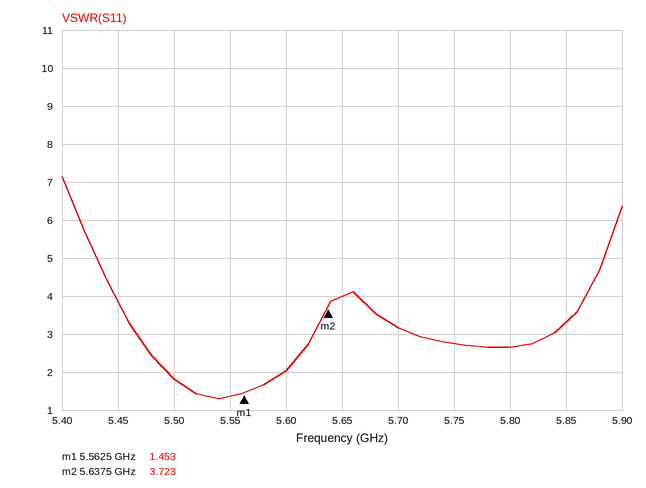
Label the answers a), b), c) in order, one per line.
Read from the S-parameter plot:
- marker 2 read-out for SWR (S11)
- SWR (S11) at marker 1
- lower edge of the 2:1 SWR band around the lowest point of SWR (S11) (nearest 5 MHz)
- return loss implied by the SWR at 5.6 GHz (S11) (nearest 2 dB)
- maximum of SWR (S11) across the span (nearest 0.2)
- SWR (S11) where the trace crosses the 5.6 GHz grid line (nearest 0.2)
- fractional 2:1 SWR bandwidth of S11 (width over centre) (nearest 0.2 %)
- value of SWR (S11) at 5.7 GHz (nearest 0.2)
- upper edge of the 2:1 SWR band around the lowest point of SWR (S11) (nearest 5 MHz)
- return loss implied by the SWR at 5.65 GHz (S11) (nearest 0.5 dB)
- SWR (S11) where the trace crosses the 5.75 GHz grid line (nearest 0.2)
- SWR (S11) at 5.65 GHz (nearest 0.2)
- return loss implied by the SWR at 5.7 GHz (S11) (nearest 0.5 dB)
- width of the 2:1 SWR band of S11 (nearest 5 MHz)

a) 3.723
b) 1.453
c) 5.495 GHz
d) 10 dB
e) 7.2
f) 2.0
g) 1.8 %
h) 3.2
i) 5.600 GHz
j) 4.5 dB
k) 2.8
l) 4.0
m) 5.5 dB
n) 105 MHz
